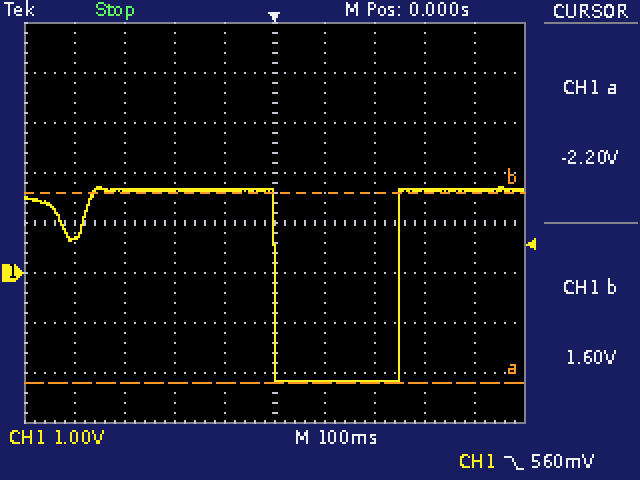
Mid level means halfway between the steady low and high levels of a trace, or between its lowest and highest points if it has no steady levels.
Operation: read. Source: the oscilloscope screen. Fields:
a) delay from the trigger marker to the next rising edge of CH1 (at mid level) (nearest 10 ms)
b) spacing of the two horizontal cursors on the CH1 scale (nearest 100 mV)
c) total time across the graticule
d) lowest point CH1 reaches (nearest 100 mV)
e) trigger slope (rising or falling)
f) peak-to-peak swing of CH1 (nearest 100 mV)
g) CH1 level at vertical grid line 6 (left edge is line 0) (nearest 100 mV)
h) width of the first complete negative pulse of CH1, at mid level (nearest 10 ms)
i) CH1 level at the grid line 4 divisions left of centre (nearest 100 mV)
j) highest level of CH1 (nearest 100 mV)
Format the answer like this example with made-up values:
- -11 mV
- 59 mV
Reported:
- 250 ms
- 3.8 V
- 1 s
- -2.2 V
- falling
- 3.9 V
- -2.2 V
- 250 ms
- 700 mV
- 1.7 V
